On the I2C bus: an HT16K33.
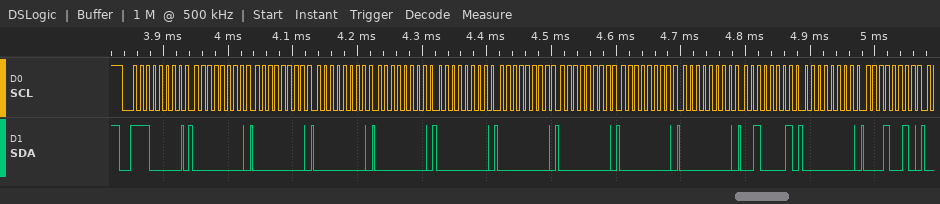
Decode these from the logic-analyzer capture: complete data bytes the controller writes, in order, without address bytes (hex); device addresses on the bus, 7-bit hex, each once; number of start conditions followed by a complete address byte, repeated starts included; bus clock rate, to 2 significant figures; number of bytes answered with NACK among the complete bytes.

00 00 00 00 00 00 00 00 00 21 00 12
0x70
1
100 kHz
0
